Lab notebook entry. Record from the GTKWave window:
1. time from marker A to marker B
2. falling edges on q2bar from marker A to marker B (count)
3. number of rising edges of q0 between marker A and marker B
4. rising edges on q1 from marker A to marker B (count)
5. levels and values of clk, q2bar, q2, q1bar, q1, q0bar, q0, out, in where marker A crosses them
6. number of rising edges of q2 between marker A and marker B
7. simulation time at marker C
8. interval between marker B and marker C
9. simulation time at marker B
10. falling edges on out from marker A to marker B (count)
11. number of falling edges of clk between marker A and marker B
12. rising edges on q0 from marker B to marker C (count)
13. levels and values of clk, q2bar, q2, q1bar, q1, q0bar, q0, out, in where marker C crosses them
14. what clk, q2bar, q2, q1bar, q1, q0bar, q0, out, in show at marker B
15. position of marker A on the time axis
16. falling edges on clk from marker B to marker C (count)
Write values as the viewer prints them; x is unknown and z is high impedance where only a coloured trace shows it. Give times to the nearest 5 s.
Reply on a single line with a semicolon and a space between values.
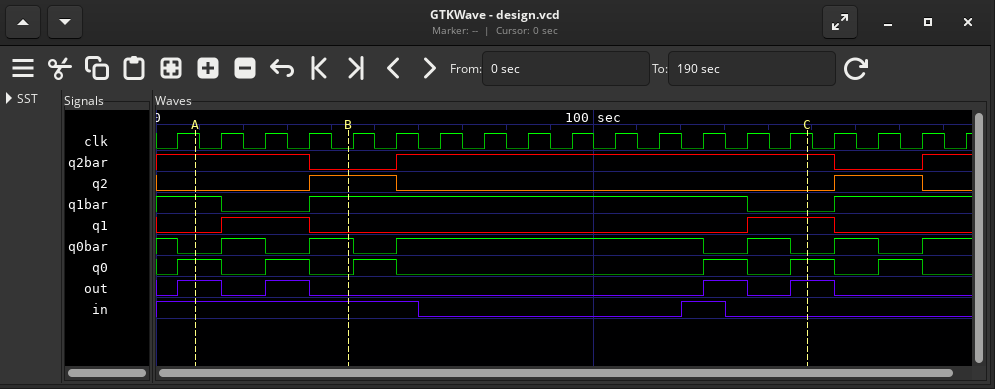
35 s; 1; 1; 1; clk=1, q2bar=1, q2=0, q1bar=1, q1=0, q0bar=0, q0=1, out=1, in=1; 1; 150 s; 105 s; 45 s; 2; 4; 3; clk=1, q2bar=1, q2=0, q1bar=0, q1=1, q0bar=0, q0=1, out=1, in=0; clk=0, q2bar=0, q2=1, q1bar=1, q1=0, q0bar=1, q0=0, out=0, in=1; 10 s; 10
